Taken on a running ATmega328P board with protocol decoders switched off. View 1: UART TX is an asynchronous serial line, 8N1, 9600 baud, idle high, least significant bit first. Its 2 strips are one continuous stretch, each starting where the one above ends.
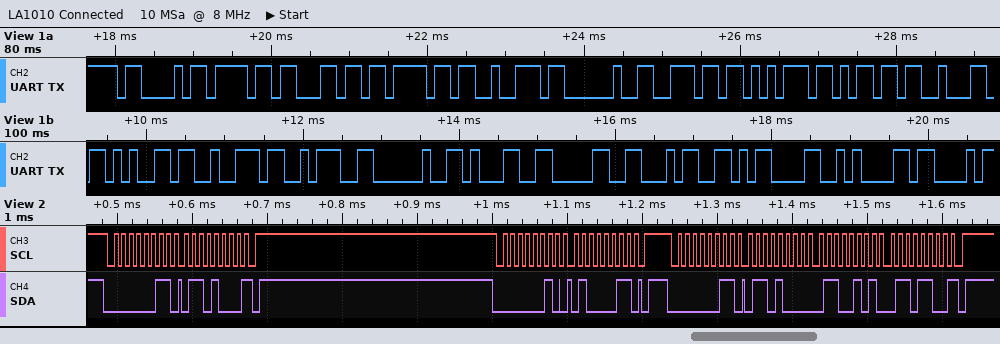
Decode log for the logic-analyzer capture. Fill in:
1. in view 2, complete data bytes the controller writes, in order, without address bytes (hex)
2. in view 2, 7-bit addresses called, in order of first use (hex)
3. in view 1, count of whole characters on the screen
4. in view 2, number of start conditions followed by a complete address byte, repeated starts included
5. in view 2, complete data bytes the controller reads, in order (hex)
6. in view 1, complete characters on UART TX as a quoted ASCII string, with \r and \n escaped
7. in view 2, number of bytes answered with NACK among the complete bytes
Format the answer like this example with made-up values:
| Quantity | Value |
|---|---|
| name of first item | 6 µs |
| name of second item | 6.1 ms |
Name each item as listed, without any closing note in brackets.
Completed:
| Quantity | Value |
|---|---|
| in view 2, complete data bytes the controller writes, in order, without address bytes | 43 |
| in view 2, 7-bit addresses called, in order of first use | 0x01 |
| in view 1, count of whole characters on the screen | 20 |
| in view 2, number of start conditions followed by a complete address byte, repeated starts included | 3 |
| in view 2, complete data bytes the controller reads, in order | 68 68 65 6C |
| in view 1, complete characters on UART TX as a quoted ASCII string, with \r and \n escaped | "Color number: 104\r\nC" |
| in view 2, number of bytes answered with NACK among the complete bytes | 2 |
